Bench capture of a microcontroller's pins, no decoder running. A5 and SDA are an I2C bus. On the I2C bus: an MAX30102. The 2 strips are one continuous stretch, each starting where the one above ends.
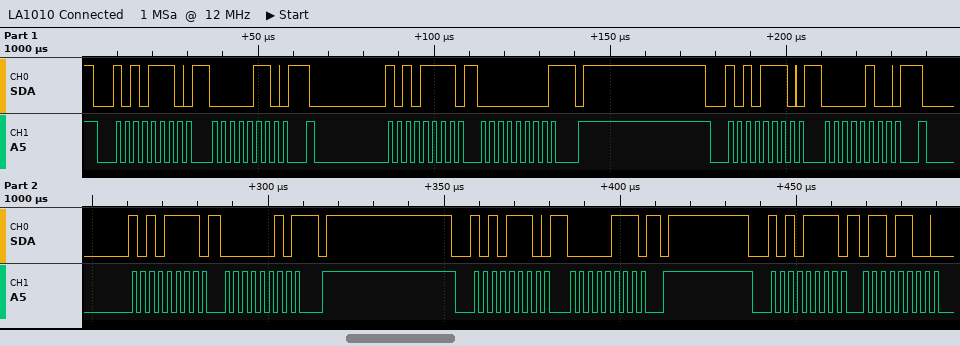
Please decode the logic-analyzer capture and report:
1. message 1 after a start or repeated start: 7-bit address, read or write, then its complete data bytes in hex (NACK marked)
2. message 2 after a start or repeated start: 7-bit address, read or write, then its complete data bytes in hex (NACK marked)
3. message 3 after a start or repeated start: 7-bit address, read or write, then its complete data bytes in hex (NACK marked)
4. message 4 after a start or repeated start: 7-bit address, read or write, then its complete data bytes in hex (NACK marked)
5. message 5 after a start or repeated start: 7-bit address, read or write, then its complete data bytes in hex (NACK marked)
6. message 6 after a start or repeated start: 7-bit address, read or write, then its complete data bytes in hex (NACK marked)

0x57 write: 06
0x57 read: 00 NACK
0x57 write: 04
0x57 read: 02 NACK
0x57 write: 07
0x57 read: 6C
